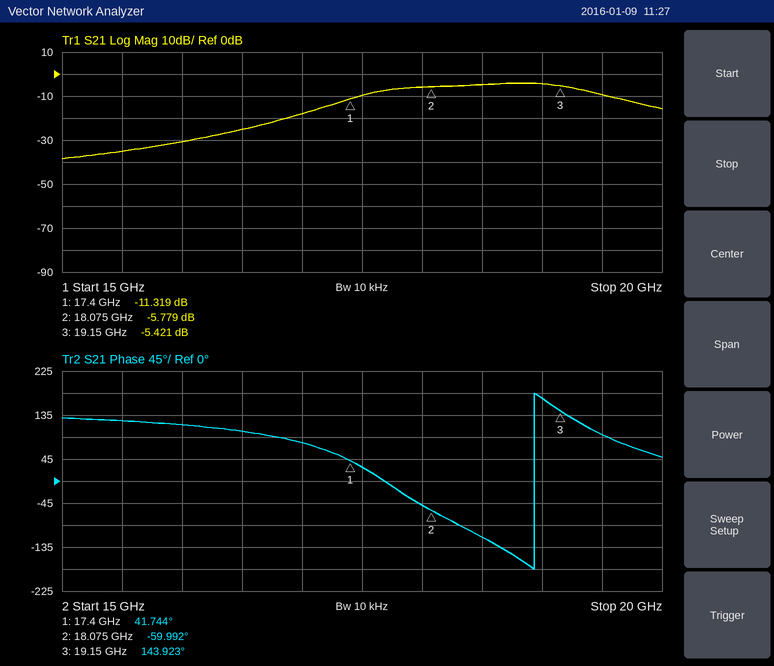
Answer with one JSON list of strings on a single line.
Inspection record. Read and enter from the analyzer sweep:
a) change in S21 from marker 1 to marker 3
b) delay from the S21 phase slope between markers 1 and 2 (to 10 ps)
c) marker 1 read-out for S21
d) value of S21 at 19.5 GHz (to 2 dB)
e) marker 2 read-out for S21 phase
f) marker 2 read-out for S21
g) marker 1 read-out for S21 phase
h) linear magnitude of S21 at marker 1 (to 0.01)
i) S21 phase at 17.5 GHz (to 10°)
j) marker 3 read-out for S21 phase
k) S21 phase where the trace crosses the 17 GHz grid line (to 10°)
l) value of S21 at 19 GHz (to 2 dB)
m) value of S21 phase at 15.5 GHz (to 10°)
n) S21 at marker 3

["5.898 dB", "420 ps", "-11.319 dB", "-10 dB", "-59.992°", "-5.779 dB", "41.744°", "0.27", "30°", "143.923°", "80°", "-4 dB", "120°", "-5.421 dB"]
